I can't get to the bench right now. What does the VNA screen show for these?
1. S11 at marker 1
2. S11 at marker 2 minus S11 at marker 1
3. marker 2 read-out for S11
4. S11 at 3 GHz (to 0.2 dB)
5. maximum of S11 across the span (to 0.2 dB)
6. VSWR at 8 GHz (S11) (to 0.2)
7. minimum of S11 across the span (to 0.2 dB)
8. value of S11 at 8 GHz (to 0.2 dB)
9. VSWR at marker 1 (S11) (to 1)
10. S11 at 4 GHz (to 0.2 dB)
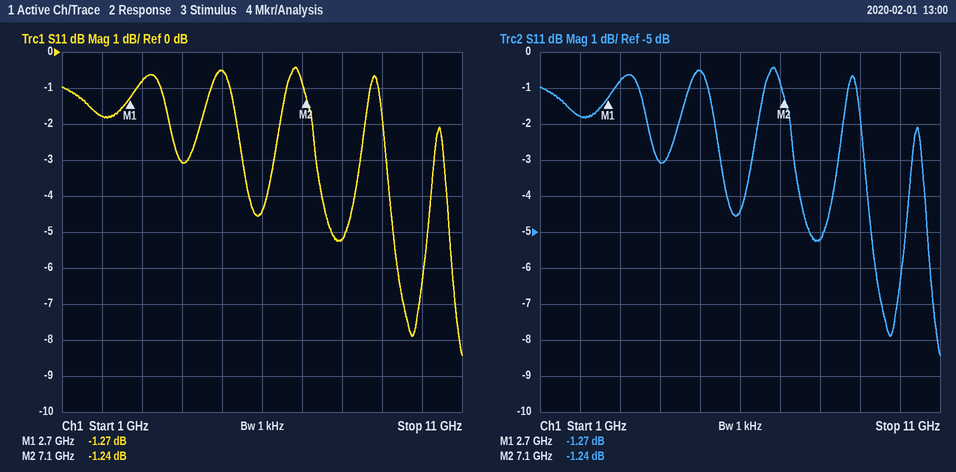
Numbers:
-1.27 dB
0.03 dB
-1.24 dB
-0.8 dB
-0.4 dB
3.4
-8.4 dB
-5.2 dB
14
-3.0 dB
